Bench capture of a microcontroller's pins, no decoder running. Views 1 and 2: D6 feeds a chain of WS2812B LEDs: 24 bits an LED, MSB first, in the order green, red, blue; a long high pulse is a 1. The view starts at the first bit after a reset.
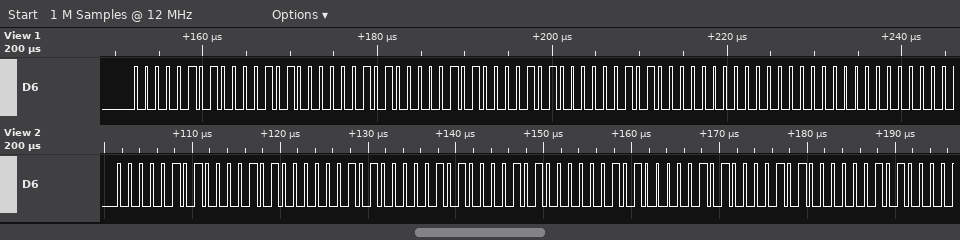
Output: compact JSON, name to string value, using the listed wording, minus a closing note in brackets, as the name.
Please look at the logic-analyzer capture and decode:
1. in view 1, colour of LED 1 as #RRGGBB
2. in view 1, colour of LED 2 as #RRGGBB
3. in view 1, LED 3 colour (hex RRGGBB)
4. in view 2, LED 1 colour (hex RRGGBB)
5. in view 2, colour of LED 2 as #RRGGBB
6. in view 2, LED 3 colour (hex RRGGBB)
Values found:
{"in view 1, colour of LED 1 as #RRGGBB": "#0A0505", "in view 1, colour of LED 2 as #RRGGBB": "#0A0505", "in view 1, LED 3 colour": "#000000", "in view 2, LED 1 colour": "#0A0505", "in view 2, colour of LED 2 as #RRGGBB": "#0A0505", "in view 2, LED 3 colour": "#0A0505"}
